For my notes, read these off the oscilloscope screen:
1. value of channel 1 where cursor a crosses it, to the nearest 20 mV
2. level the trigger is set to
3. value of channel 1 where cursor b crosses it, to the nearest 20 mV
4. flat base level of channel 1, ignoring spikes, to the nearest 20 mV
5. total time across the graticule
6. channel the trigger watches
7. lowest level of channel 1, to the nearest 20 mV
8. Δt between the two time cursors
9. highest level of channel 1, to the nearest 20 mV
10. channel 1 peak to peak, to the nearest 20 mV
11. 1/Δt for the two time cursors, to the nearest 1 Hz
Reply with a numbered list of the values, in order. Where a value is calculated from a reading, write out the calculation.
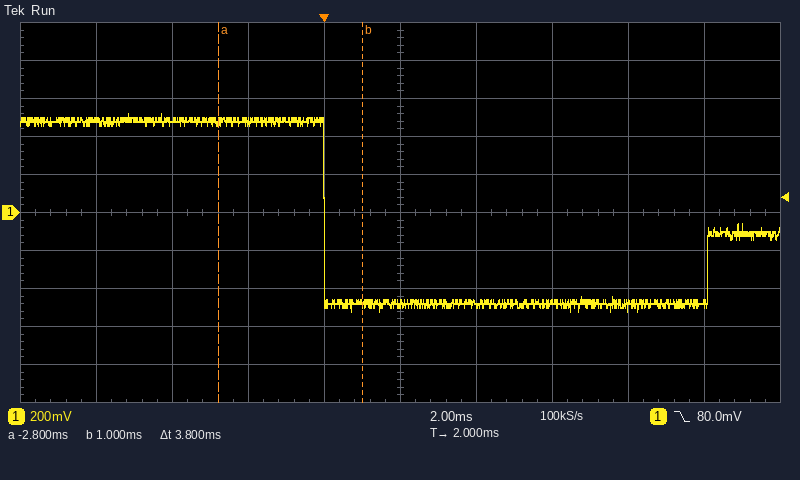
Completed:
1. 480 mV
2. 80.0 mV
3. -480 mV
4. -480 mV
5. 20 ms
6. channel 1
7. -520 mV
8. 3.8 ms
9. 520 mV
10. 520 mV − (-520 mV) = 1.04 V
11. 1 / 3.8 ms ≈ 263 Hz
